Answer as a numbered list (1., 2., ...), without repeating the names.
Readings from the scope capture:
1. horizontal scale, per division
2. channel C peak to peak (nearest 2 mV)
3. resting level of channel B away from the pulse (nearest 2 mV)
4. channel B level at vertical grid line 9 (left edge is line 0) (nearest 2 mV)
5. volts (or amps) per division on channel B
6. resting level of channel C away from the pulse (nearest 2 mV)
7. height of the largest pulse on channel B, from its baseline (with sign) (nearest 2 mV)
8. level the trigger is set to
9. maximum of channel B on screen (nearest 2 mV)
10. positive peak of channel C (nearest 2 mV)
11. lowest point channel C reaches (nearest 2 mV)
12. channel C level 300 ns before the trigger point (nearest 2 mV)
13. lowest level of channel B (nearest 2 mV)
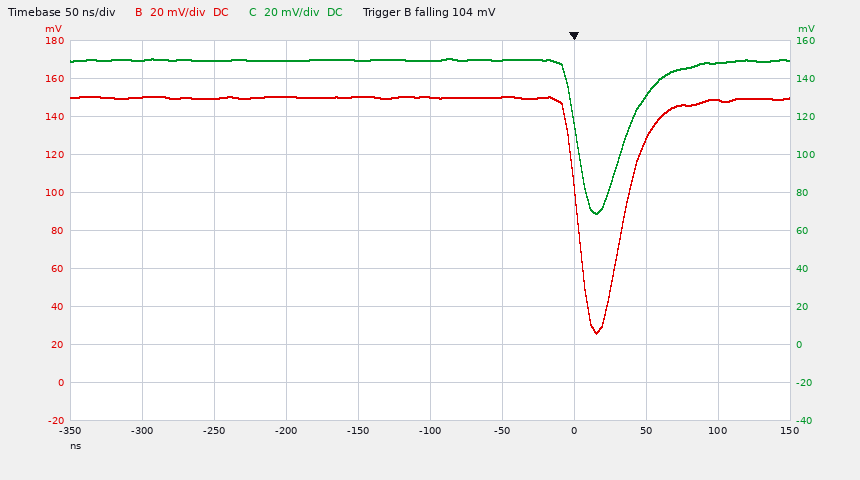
1. 50 ns
2. 82 mV
3. 150 mV
4. 148 mV
5. 20 mV
6. 150 mV
7. -124 mV
8. 104 mV
9. 150 mV
10. 150 mV
11. 68 mV
12. 150 mV
13. 26 mV
